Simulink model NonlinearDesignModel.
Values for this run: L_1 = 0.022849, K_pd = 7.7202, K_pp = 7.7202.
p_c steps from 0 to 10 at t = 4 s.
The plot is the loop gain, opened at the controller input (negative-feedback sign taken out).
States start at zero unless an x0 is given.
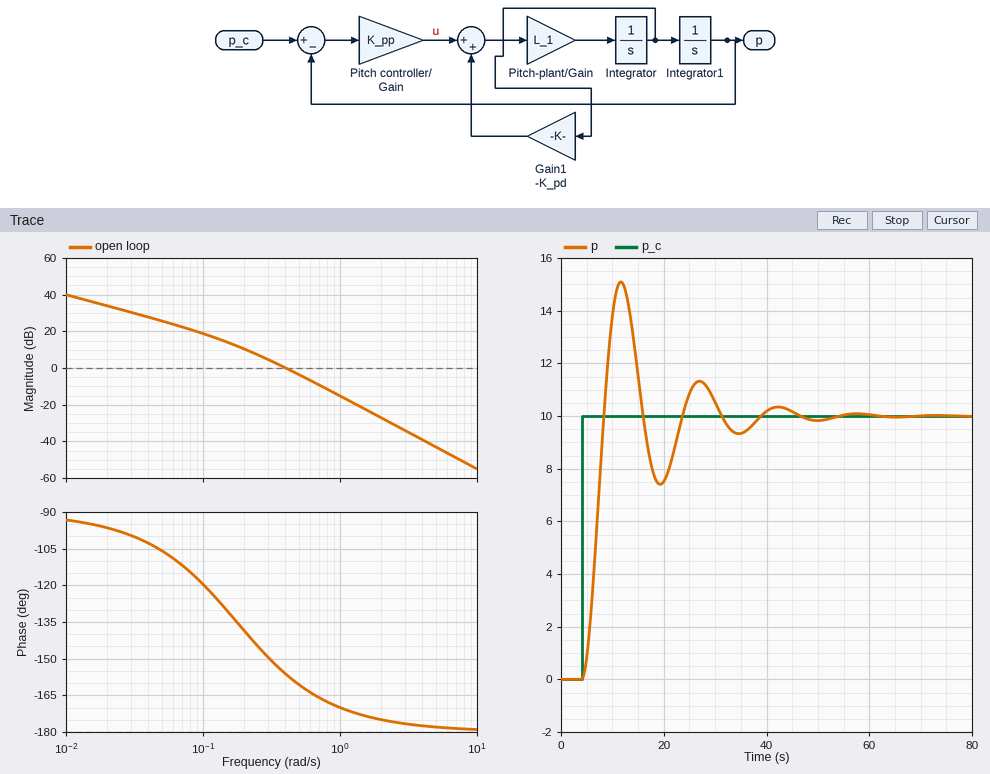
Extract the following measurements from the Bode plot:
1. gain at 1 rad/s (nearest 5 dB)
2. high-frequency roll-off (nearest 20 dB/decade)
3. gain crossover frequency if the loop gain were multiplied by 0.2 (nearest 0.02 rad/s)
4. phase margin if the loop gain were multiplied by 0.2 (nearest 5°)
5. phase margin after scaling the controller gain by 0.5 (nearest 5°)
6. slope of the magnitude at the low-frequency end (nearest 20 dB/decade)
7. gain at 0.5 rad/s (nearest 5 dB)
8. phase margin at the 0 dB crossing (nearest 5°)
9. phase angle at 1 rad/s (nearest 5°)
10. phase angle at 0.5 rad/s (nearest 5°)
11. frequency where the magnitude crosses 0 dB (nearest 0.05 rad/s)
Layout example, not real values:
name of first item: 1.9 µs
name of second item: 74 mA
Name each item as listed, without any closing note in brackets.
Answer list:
gain at 1 rad/s: -15 dB
high-frequency roll-off: -40 dB/decade
gain crossover frequency if the loop gain were multiplied by 0.2: 0.16 rad/s
phase margin if the loop gain were multiplied by 0.2: 50°
phase margin after scaling the controller gain by 0.5: 35°
slope of the magnitude at the low-frequency end: -20 dB/decade
gain at 0.5 rad/s: -5 dB
phase margin at the 0 dB crossing: 25°
phase angle at 1 rad/s: -170°
phase angle at 0.5 rad/s: -160°
frequency where the magnitude crosses 0 dB: 0.40 rad/s
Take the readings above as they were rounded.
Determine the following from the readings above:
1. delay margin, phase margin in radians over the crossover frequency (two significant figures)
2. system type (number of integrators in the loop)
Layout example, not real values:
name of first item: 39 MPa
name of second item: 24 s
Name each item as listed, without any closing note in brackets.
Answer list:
delay margin, phase margin in radians over the crossover frequency: 1.1 s
system type: 1
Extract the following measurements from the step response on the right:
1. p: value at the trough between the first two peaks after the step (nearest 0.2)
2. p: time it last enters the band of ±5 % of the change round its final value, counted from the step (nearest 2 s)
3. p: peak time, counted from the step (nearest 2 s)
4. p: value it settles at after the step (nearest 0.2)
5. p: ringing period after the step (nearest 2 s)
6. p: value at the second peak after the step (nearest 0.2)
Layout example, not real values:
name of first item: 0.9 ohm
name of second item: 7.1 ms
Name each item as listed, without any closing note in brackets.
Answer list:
p: value at the trough between the first two peaks after the step: 7.4
p: time it last enters the band of ±5 % of the change round its final value, counted from the step: 32 s
p: peak time, counted from the step: 8 s
p: value it settles at after the step: 10.0
p: ringing period after the step: 16 s
p: value at the second peak after the step: 11.4
